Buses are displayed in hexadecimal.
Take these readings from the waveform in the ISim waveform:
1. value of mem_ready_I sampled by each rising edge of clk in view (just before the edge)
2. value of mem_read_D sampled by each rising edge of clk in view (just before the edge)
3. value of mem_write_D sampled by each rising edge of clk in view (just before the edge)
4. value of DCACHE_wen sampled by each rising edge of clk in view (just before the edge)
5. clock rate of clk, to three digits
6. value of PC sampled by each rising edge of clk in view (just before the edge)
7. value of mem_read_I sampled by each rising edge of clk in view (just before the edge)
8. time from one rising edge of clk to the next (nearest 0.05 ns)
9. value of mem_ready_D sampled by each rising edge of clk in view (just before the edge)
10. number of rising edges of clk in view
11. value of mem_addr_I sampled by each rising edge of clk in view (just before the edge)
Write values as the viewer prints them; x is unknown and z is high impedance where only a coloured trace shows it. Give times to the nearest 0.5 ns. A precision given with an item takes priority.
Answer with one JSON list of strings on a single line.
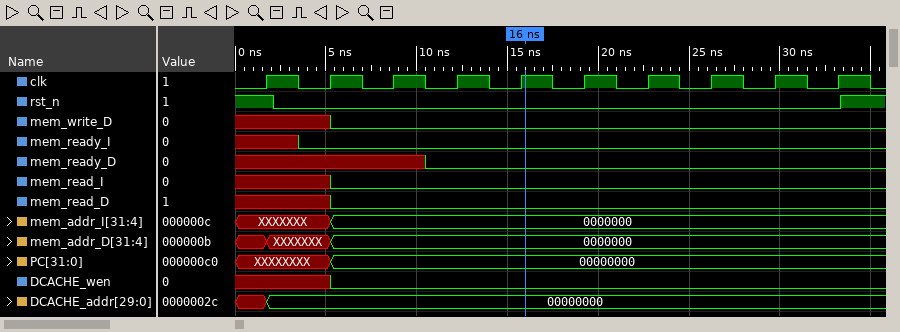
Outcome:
["x 0 0 0 0 0 0 0 0 0", "x x 0 0 0 0 0 0 0 0", "x x 0 0 0 0 0 0 0 0", "x x 0 0 0 0 0 0 0 0", "286 MHz", "XXXXXXXX, XXXXXXXX, 00000000, 00000000, 00000000, 00000000, 00000000, 00000000, 00000000, 00000000", "x x 0 0 0 0 0 0 0 0", "3.5 ns", "x x x 0 0 0 0 0 0 0", "10", "XXXXXXX, XXXXXXX, 0000000, 0000000, 0000000, 0000000, 0000000, 0000000, 0000000, 0000000"]
